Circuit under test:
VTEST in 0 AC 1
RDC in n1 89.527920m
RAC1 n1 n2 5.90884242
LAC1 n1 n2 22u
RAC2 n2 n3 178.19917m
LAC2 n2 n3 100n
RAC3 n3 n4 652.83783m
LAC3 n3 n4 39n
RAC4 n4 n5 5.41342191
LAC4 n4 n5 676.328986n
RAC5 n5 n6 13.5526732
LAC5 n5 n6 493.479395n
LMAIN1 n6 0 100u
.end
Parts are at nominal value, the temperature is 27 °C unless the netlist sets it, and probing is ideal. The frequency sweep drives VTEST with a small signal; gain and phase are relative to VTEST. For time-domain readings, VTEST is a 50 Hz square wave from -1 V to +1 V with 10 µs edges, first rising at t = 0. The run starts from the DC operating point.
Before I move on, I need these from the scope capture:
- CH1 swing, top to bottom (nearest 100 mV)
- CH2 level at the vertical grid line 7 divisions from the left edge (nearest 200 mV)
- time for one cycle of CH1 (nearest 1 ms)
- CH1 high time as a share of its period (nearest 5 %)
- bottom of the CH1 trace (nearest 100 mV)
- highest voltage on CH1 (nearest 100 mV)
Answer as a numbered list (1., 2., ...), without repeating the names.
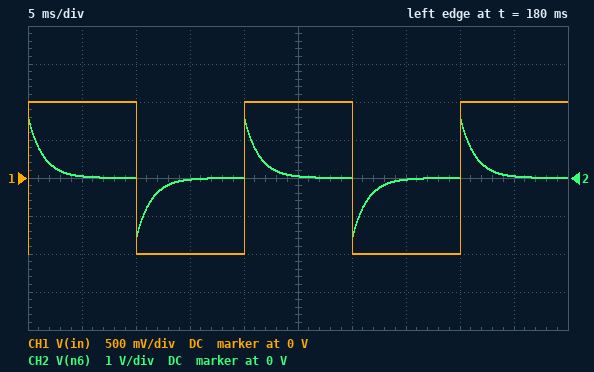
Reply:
1. 2.0 V
2. 0 V
3. 20 ms
4. 50 %
5. -1.0 V
6. 1.0 V
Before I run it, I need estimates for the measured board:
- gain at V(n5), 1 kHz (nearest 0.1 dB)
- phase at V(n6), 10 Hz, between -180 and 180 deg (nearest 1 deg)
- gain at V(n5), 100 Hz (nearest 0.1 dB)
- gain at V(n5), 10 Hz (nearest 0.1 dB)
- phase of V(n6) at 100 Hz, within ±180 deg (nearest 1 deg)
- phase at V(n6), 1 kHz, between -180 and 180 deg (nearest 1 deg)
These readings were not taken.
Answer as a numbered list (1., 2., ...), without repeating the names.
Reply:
1. -1.8 dB
2. 85 deg
3. -5.5 dB
4. -23.1 dB
5. 49 deg
6. 7 deg
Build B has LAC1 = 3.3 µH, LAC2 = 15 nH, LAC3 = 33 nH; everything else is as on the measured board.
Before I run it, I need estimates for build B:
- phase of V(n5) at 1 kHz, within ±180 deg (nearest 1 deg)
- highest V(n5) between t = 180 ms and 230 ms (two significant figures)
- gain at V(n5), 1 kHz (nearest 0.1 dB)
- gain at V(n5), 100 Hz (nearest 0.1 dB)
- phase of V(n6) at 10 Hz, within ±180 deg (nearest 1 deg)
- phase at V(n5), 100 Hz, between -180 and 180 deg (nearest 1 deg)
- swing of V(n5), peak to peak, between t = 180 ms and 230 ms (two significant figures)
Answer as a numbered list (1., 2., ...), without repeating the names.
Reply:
1. 8 deg
2. 1.9 V
3. -0.4 dB
4. -4.9 dB
5. 86 deg
6. 54 deg
7. 3.8 V
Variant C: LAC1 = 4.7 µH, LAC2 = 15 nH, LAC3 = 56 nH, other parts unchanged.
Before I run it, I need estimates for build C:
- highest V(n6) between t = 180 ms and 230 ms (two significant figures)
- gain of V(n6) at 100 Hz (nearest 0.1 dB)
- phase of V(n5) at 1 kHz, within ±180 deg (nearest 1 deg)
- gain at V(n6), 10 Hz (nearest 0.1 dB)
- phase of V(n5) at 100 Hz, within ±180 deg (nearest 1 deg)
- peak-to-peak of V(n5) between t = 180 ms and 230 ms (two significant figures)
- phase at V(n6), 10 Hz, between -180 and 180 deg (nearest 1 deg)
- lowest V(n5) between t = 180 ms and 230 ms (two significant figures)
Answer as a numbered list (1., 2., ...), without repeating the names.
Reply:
1. 1.9 V
2. -5.0 dB
3. 8 deg
4. -23.1 dB
5. 53 deg
6. 3.8 V
7. 86 deg
8. -1.9 V
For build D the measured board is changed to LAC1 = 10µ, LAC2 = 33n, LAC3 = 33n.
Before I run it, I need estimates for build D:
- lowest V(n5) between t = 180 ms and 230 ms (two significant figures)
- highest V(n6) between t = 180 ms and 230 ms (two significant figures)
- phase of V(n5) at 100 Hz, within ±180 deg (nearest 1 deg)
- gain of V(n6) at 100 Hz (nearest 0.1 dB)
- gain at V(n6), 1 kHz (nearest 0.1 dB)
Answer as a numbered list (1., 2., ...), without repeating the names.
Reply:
1. -1.8 V
2. 1.8 V
3. 52 deg
4. -5.1 dB
5. -1.0 dB
